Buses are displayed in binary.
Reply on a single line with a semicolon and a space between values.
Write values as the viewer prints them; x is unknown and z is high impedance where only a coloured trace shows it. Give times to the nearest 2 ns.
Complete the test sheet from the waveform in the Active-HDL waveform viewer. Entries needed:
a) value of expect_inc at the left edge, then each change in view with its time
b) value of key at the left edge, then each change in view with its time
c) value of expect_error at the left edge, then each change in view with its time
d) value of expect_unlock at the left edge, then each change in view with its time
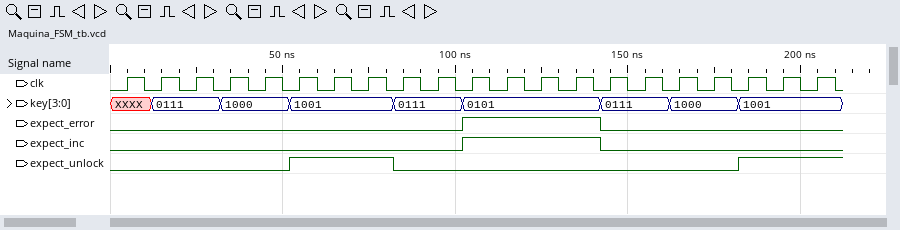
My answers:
0, 1 at 102 ns, 0 at 142 ns; XXXX, 0111 at 12 ns, 1000 at 32 ns, 1001 at 52 ns, 0111 at 82 ns, 0101 at 102 ns, 0111 at 142 ns, 1000 at 162 ns, 1001 at 182 ns; 0, 1 at 102 ns, 0 at 142 ns; 0, 1 at 52 ns, 0 at 82 ns, 1 at 182 ns
